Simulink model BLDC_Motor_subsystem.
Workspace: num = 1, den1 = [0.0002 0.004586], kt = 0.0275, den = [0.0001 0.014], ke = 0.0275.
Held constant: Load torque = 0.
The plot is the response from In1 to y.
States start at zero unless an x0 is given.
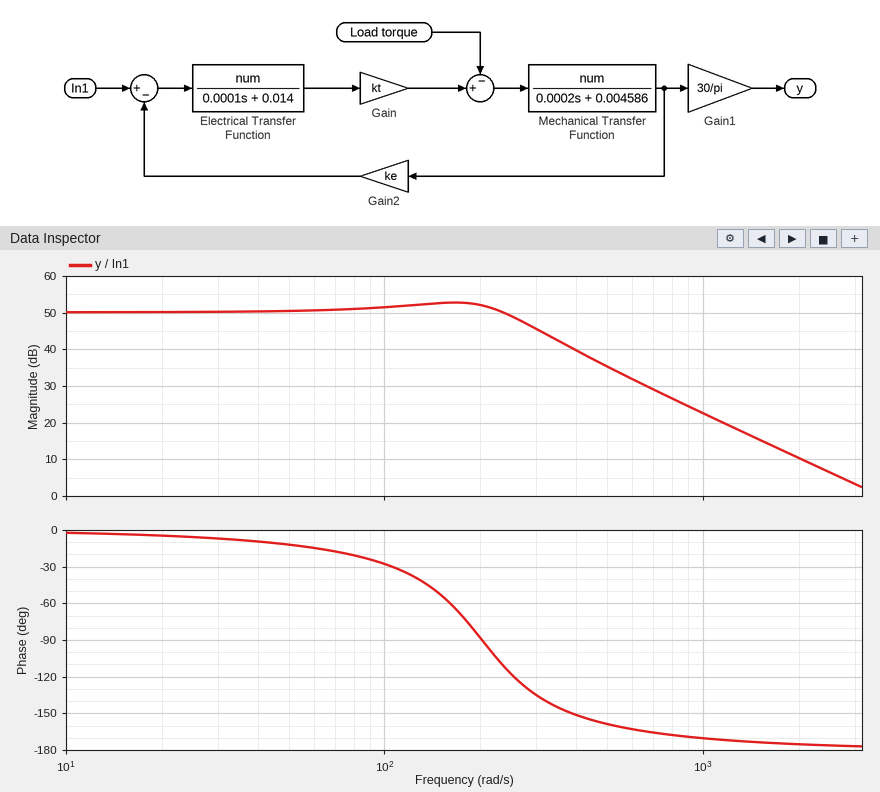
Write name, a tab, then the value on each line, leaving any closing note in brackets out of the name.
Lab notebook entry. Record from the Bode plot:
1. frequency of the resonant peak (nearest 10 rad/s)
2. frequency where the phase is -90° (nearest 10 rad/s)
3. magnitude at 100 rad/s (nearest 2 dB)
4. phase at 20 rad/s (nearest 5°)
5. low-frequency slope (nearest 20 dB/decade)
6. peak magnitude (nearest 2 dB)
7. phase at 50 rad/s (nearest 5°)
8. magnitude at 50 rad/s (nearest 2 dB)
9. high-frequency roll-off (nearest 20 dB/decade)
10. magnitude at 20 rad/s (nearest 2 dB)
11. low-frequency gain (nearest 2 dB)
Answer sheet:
frequency of the resonant peak	160 rad/s
frequency where the phase is -90°	200 rad/s
magnitude at 100 rad/s	52 dB
phase at 20 rad/s	-5°
low-frequency slope	0 dB/decade
peak magnitude	52 dB
phase at 50 rad/s	-10°
magnitude at 50 rad/s	50 dB
high-frequency roll-off	-40 dB/decade
magnitude at 20 rad/s	50 dB
low-frequency gain	50 dB
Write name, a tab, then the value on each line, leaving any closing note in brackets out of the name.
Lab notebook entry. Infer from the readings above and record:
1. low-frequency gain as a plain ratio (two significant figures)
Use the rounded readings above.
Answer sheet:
low-frequency gain as a plain ratio	320
